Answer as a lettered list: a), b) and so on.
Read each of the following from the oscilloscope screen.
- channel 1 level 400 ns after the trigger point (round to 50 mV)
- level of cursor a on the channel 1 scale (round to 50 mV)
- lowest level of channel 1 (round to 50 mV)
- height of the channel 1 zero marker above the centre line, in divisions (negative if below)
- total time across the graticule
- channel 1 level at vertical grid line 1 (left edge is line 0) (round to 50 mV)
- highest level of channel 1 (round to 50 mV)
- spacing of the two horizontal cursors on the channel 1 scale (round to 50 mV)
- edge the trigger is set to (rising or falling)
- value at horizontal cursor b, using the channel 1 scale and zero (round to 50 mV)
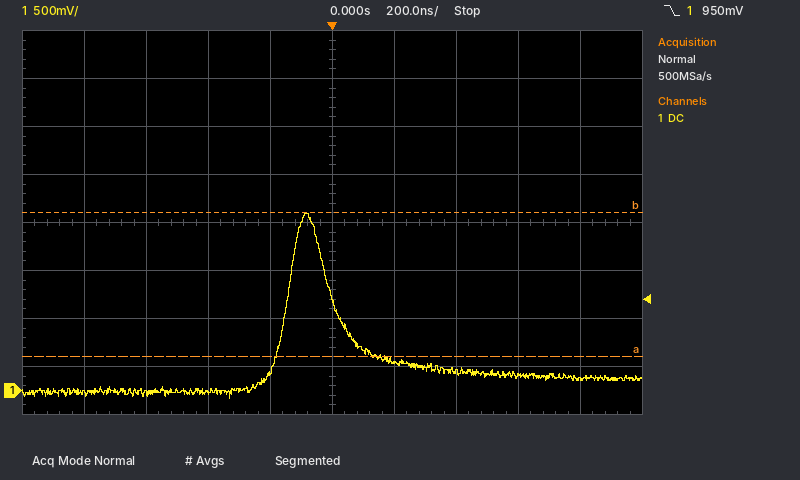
a) 200 mV
b) 350 mV
c) -100 mV
d) -3.5 div
e) 2 µs
f) -50 mV
g) 1.85 V
h) 1.50 V
i) falling
j) 1.85 V
